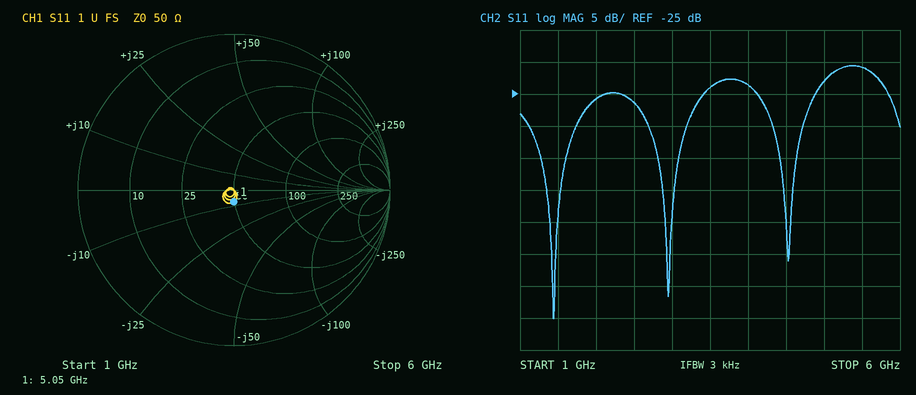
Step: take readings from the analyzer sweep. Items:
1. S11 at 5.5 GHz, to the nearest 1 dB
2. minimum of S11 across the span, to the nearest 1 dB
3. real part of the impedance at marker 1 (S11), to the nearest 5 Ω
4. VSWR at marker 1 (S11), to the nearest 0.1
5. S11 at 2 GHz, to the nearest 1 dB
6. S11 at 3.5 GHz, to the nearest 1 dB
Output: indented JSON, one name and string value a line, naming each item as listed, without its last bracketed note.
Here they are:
{
  "S11 at 5.5 GHz, to the nearest 1 dB": "-21 dB",
  "minimum of S11 across the span, to the nearest 1 dB": "-60 dB",
  "real part of the impedance at marker 1 (S11), to the nearest 5 Ω": "50 Ω",
  "VSWR at marker 1 (S11), to the nearest 0.1": "1.2",
  "S11 at 2 GHz, to the nearest 1 dB": "-26 dB",
  "S11 at 3.5 GHz, to the nearest 1 dB": "-24 dB"
}
